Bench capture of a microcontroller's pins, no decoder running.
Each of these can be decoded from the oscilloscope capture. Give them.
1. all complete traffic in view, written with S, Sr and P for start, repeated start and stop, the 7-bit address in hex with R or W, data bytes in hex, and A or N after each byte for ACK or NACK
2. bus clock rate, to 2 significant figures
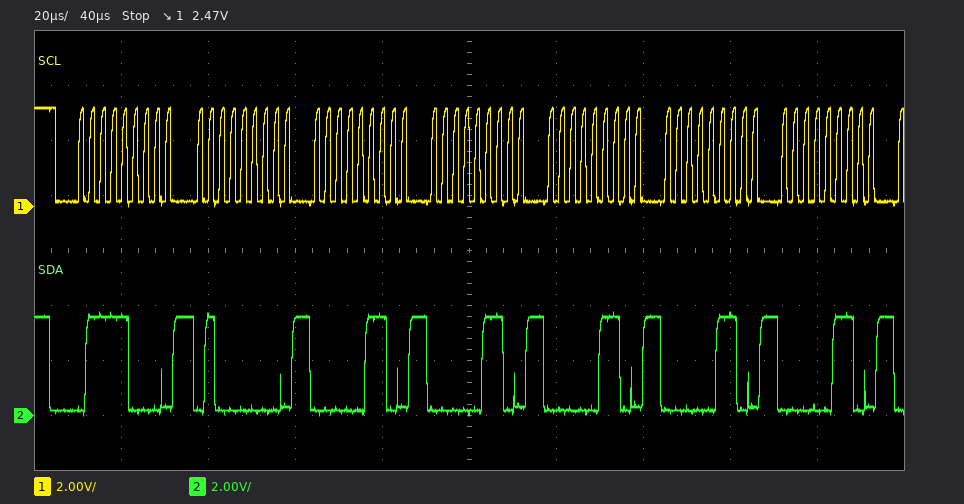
S 3CW A 40 A 06 A 06 A 06 A 06 A 06 A
400 kHz
